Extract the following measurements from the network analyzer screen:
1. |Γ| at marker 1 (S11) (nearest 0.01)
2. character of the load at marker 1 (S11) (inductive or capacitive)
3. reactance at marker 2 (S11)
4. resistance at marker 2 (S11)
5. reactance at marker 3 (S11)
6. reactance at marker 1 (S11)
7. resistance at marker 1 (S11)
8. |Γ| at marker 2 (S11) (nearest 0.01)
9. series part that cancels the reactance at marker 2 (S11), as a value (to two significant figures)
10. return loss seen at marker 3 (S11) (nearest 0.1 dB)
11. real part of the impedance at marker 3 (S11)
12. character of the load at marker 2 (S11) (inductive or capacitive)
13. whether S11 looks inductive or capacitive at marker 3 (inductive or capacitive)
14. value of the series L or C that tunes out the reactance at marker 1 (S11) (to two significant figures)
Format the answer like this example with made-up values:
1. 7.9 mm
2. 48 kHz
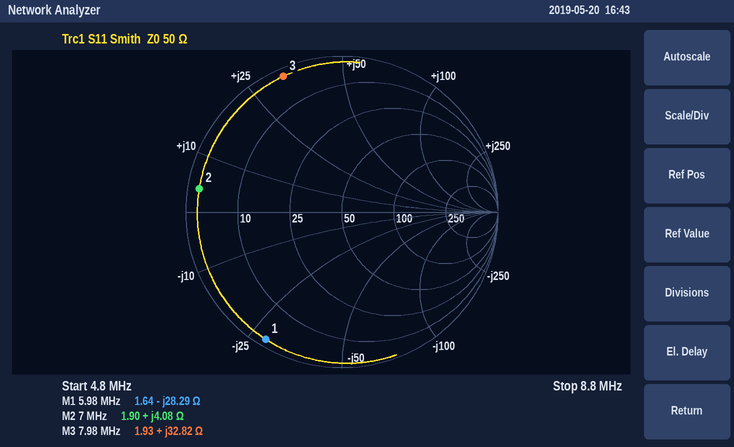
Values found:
1. 0.95
2. capacitive
3. +4.08 Ω
4. 1.90 Ω
5. +32.82 Ω
6. -28.29 Ω
7. 1.64 Ω
8. 0.93
9. 5.6 nF
10. 0.5 dB
11. 1.93 Ω
12. inductive
13. inductive
14. 750 nH
